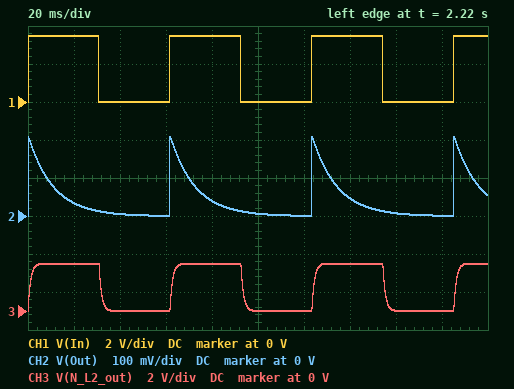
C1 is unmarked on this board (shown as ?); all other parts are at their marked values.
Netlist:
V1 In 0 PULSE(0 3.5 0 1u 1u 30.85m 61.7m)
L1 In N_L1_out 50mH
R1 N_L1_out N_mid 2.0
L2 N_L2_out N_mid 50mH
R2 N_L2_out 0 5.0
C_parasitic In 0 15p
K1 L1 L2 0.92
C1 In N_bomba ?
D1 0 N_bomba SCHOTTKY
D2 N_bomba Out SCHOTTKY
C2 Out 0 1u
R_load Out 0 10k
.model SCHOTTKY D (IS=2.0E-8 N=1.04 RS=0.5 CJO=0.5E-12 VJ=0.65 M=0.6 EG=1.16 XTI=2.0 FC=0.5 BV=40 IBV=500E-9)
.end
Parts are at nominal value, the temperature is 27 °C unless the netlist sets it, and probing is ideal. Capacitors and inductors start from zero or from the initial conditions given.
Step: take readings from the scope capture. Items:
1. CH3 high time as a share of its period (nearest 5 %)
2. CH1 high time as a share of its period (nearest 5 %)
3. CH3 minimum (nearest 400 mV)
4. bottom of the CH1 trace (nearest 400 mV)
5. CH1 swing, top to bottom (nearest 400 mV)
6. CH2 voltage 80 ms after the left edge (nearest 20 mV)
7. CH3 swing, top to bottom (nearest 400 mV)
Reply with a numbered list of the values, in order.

1. 50 %
2. 50 %
3. 0 V
4. 0 V
5. 3.6 V
6. 40 mV
7. 2.4 V
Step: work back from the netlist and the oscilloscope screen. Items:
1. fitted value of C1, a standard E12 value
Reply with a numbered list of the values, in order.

1. 68 nF
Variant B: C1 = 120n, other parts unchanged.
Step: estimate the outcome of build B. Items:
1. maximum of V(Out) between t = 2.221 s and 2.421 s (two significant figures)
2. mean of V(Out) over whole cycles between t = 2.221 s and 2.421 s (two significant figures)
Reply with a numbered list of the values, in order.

1. 350 mV
2. 65 mV
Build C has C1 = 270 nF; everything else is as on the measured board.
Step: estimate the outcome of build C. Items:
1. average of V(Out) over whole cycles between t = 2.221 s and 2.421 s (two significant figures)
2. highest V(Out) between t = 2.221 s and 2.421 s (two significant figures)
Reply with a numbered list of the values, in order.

1. 140 mV
2. 680 mV
